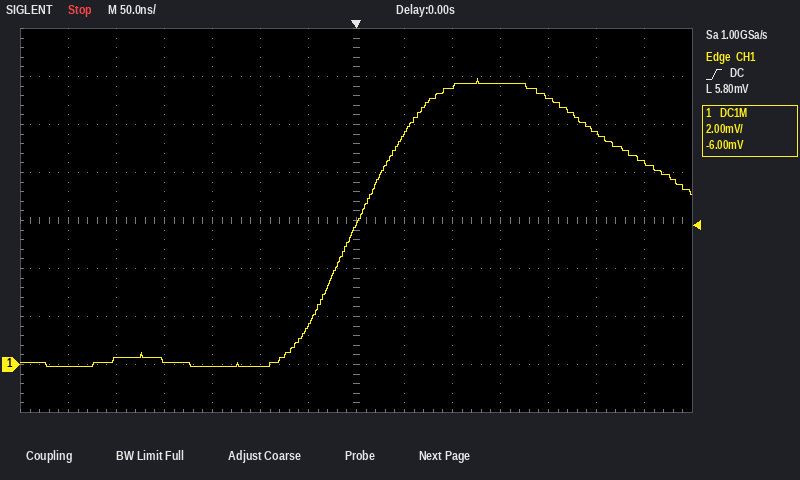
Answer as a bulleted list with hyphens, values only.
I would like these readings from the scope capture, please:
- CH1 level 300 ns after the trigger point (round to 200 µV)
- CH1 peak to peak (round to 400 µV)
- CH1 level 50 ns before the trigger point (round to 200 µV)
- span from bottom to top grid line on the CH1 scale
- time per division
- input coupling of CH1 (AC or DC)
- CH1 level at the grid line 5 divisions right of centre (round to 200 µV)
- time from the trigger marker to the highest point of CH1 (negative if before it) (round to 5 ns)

- 8.4 mV
- 12.0 mV
- 1.6 mV
- 16 mV
- 50 ns
- DC
- 9.6 mV
- +125 ns
